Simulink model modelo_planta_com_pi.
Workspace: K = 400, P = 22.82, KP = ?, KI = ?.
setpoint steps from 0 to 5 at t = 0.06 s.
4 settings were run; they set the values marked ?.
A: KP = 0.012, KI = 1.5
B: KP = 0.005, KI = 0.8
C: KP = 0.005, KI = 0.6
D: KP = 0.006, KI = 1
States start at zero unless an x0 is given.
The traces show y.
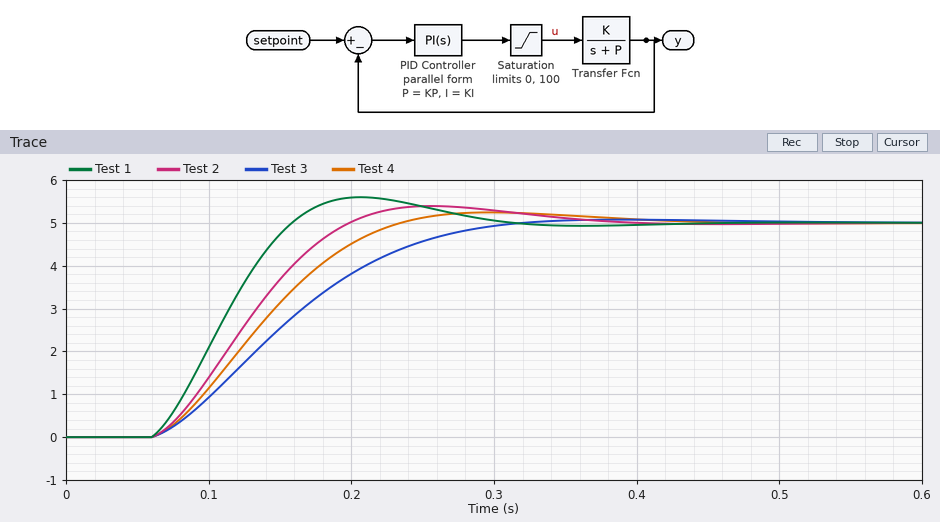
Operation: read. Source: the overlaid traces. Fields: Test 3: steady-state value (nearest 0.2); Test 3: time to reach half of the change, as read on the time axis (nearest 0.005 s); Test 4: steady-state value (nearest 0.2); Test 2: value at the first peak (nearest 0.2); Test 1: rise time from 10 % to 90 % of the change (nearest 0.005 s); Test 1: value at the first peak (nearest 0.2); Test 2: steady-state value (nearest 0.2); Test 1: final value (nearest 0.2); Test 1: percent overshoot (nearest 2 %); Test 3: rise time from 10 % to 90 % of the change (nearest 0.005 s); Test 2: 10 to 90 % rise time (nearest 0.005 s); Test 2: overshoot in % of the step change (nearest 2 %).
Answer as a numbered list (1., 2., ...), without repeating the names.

1. 5.0
2. 0.150 s
3. 5.0
4. 5.4
5. 0.070 s
6. 5.6
7. 5.0
8. 5.0
9. 12 %
10. 0.160 s
11. 0.095 s
12. 8 %
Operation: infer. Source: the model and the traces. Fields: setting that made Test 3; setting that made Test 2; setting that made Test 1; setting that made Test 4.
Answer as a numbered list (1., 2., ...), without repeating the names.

1. C
2. D
3. A
4. B
